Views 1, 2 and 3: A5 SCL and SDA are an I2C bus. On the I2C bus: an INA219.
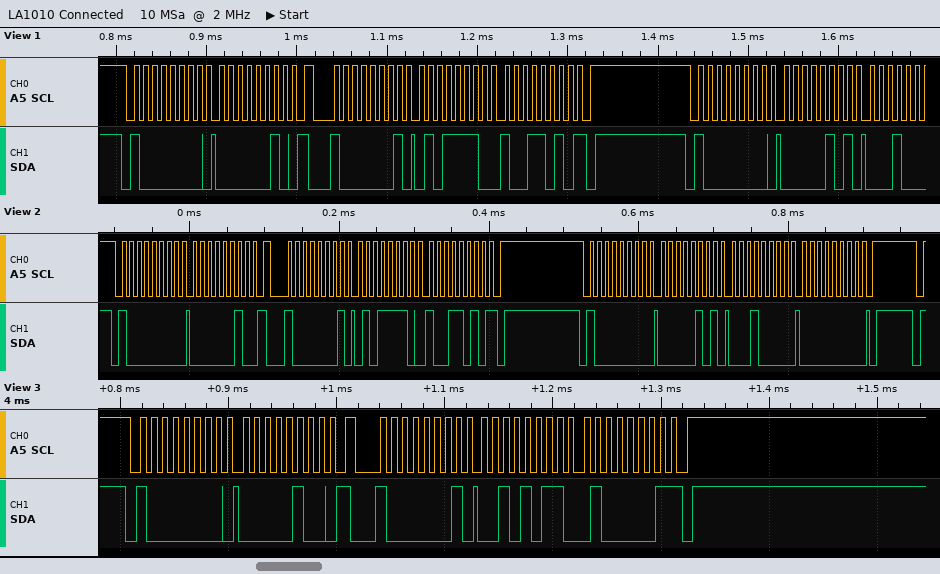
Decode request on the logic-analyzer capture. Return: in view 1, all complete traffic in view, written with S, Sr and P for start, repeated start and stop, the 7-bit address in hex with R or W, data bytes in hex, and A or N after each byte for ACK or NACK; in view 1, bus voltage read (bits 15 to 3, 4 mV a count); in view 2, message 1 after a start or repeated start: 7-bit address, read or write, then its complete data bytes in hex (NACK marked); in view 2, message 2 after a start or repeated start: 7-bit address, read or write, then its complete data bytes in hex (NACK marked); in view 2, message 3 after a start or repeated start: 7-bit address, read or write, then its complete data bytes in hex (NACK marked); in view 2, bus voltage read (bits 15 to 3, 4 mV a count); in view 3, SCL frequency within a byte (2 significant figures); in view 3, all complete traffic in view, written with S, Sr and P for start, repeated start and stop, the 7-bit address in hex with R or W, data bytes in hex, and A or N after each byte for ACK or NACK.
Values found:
S 40W A 02 A Sr 40R A 5E A 9A N P S 40W A 05 A
12.108 V
0x40 write: 02
0x40 read: 5E 9A NACK
0x40 write: 05 10 00
12.108 V
100 kHz
S 40W A 04 A Sr 40R A 2B A 41 N P
